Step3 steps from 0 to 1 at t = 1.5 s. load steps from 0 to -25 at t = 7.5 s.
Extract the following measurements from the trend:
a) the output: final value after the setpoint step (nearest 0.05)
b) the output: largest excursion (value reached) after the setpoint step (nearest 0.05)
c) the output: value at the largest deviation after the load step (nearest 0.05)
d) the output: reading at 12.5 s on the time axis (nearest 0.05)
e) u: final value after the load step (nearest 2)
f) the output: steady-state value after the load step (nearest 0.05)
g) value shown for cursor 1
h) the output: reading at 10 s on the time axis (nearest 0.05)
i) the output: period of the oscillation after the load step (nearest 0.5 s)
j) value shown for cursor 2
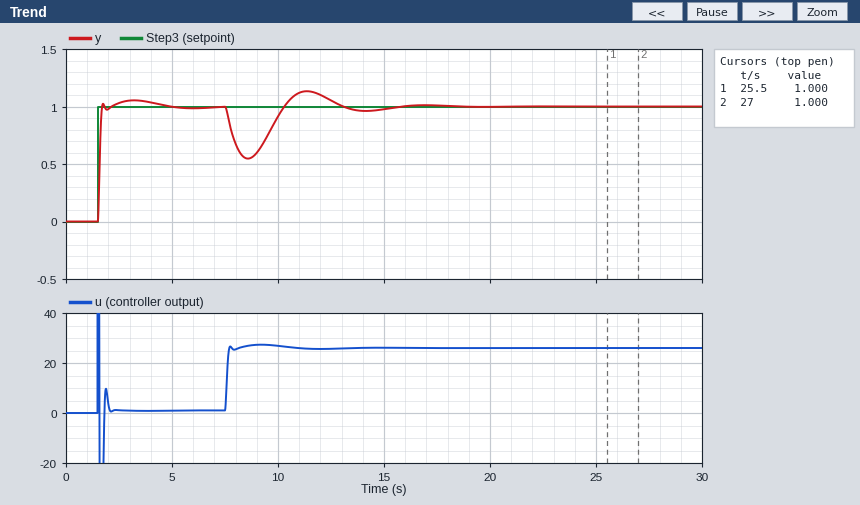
1.00
1.05
0.55
1.05
26
1.00
1.000
0.90
5.5 s
1.000
